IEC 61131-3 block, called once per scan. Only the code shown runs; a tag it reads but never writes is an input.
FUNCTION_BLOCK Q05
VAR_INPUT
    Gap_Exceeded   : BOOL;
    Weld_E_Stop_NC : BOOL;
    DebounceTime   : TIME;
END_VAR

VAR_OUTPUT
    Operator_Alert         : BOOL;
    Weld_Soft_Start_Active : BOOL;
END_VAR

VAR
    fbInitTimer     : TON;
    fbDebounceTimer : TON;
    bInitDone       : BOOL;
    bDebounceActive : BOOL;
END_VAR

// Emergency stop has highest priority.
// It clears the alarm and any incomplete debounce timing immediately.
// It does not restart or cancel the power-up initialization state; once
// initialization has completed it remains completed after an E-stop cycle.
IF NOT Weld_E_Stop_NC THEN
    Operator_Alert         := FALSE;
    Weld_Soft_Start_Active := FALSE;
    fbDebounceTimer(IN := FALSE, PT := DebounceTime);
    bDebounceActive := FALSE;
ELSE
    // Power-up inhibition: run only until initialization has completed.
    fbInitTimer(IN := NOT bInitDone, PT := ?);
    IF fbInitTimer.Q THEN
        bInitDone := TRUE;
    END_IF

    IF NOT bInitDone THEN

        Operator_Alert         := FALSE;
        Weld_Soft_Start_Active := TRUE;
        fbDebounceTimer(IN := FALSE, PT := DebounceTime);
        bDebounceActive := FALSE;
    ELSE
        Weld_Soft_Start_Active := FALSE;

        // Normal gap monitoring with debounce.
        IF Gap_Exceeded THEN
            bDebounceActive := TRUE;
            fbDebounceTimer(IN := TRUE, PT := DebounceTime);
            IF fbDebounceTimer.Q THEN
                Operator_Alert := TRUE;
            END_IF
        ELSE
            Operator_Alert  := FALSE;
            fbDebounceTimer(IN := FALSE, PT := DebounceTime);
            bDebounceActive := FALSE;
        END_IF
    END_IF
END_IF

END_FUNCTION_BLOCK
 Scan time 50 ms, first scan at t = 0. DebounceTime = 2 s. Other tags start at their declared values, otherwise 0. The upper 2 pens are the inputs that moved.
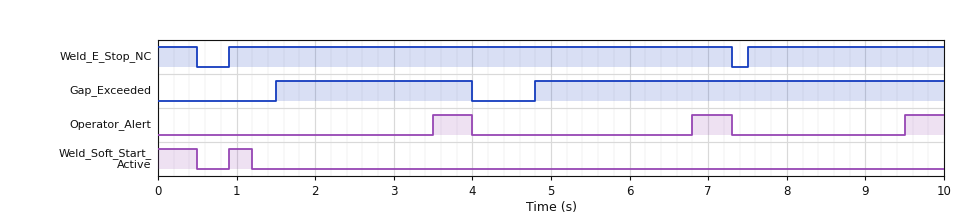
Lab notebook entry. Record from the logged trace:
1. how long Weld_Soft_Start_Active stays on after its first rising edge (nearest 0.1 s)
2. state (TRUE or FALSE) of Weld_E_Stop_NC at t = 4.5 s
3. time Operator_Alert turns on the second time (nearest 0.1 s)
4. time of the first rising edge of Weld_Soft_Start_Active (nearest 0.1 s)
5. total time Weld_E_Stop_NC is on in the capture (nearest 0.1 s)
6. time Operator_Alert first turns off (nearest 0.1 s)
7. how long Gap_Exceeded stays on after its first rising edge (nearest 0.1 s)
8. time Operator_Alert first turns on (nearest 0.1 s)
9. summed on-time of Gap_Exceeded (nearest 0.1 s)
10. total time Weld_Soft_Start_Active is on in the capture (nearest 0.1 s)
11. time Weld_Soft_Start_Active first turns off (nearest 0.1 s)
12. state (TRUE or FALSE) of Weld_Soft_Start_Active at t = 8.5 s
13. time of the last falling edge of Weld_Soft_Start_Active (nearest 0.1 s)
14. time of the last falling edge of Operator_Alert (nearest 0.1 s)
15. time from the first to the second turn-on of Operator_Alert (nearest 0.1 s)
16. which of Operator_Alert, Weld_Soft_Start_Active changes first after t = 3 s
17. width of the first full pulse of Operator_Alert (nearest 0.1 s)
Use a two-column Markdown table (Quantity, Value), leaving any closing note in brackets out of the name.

| Quantity | Value |
|---|---|
| how long Weld_Soft_Start_Active stays on after its first rising edge | 0.3 s |
| state (TRUE or FALSE) of Weld_E_Stop_NC at t = 4.5 s | TRUE |
| time Operator_Alert turns on the second time | 6.8 s |
| time of the first rising edge of Weld_Soft_Start_Active | 0.9 s |
| total time Weld_E_Stop_NC is on in the capture | 9.4 s |
| time Operator_Alert first turns off | 4.0 s |
| how long Gap_Exceeded stays on after its first rising edge | 2.5 s |
| time Operator_Alert first turns on | 3.5 s |
| summed on-time of Gap_Exceeded | 7.7 s |
| total time Weld_Soft_Start_Active is on in the capture | 0.8 s |
| time Weld_Soft_Start_Active first turns off | 0.5 s |
| state (TRUE or FALSE) of Weld_Soft_Start_Active at t = 8.5 s | FALSE |
| time of the last falling edge of Weld_Soft_Start_Active | 1.2 s |
| time of the last falling edge of Operator_Alert | 7.3 s |
| time from the first to the second turn-on of Operator_Alert | 3.3 s |
| which of Operator_Alert, Weld_Soft_Start_Active changes first after t = 3 s | Operator_Alert |
| width of the first full pulse of Operator_Alert | 0.5 s |
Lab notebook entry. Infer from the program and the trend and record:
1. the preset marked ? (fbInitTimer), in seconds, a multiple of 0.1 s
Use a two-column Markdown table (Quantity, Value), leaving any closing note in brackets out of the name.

| Quantity | Value |
|---|---|
| the preset marked ? (fbInitTimer), in seconds, a multiple of 0.1 s | 1.2 s |
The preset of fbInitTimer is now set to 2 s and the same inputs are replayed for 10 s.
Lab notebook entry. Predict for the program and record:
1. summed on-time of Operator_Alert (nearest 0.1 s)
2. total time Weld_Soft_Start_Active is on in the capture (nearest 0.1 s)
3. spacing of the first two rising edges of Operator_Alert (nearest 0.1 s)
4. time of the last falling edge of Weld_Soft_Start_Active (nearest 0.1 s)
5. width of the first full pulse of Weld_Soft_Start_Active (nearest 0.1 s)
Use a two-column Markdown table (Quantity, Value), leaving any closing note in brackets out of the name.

| Quantity | Value |
|---|---|
| summed on-time of Operator_Alert | 1.0 s |
| total time Weld_Soft_Start_Active is on in the capture | 1.6 s |
| spacing of the first two rising edges of Operator_Alert | 2.7 s |
| time of the last falling edge of Weld_Soft_Start_Active | 2.0 s |
| width of the first full pulse of Weld_Soft_Start_Active | 1.1 s |
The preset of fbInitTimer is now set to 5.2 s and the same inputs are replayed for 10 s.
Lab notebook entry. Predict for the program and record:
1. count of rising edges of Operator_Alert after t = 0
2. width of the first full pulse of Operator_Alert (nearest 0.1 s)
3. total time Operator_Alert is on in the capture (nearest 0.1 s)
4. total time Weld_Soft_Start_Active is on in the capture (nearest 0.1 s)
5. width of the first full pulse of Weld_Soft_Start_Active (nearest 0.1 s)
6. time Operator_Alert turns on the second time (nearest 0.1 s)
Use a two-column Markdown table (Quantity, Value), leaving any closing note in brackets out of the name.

| Quantity | Value |
|---|---|
| count of rising edges of Operator_Alert after t = 0 | 2 |
| width of the first full pulse of Operator_Alert | 0.1 s |
| total time Operator_Alert is on in the capture | 0.6 s |
| total time Weld_Soft_Start_Active is on in the capture | 4.8 s |
| width of the first full pulse of Weld_Soft_Start_Active | 4.3 s |
| time Operator_Alert turns on the second time | 9.5 s |
